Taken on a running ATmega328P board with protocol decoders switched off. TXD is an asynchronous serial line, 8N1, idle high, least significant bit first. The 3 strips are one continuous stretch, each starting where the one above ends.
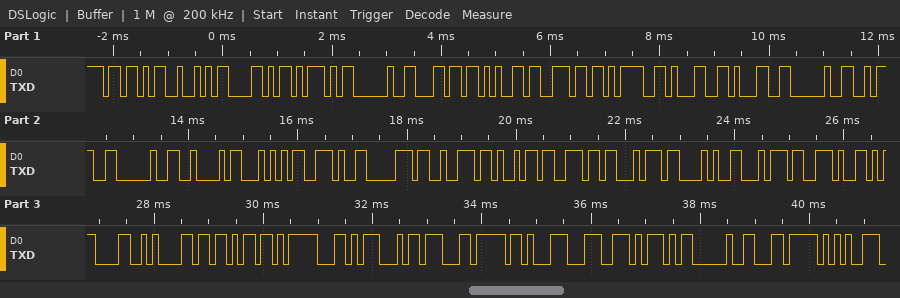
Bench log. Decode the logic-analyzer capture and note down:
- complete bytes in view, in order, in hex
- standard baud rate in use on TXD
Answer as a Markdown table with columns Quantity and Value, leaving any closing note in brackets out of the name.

| Quantity | Value |
|---|---|
| complete bytes in view, in order, in hex | 0x5B 0x52 0x58 0x5D 0x20 0x6C 0x65 0x6E 0x3D 0x31 0x31 0x20 0x3A 0x20 0x42 0x54 0x2E 0x70 0x72 0x69 0x6E 0x74 0x28 0x74 0x2E 0x0D 0x0A 0x5B 0xEB 0xAC 0xB4 0xEC 0x8B 0x9C 0x5D 0x20 0xEC 0x95 |
| standard baud rate in use on TXD | 9600 baud |
